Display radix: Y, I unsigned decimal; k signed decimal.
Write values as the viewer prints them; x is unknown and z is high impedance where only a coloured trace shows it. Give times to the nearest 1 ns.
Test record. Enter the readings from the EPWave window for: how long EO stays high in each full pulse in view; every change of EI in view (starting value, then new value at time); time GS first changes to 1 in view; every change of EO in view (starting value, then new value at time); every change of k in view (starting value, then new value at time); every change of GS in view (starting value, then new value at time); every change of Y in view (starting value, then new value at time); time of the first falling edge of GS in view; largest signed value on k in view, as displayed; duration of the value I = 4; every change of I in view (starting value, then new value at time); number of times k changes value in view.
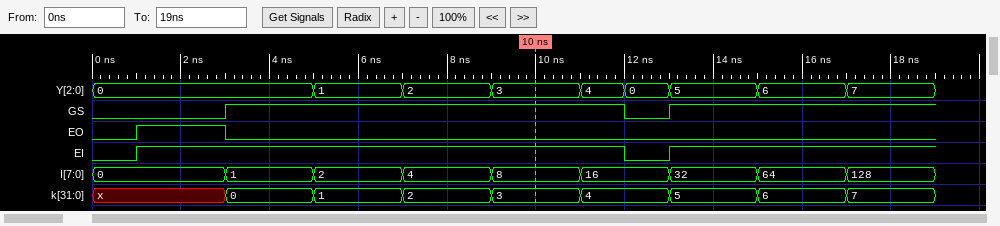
2 ns
0, 1 at 1 ns, 0 at 12 ns, 1 at 13 ns
3 ns
0, 1 at 1 ns, 0 at 3 ns
x, 0 at 3 ns, 1 at 5 ns, 2 at 7 ns, 3 at 9 ns, 4 at 11 ns, 5 at 13 ns, 6 at 15 ns, 7 at 17 ns
0, 1 at 3 ns, 0 at 12 ns, 1 at 13 ns
0, 1 at 5 ns, 2 at 7 ns, 3 at 9 ns, 4 at 11 ns, 0 at 12 ns, 5 at 13 ns, 6 at 15 ns, 7 at 17 ns
12 ns
7
2 ns
0, 1 at 3 ns, 2 at 5 ns, 4 at 7 ns, 8 at 9 ns, 16 at 11 ns, 32 at 13 ns, 64 at 15 ns, 128 at 17 ns
8
